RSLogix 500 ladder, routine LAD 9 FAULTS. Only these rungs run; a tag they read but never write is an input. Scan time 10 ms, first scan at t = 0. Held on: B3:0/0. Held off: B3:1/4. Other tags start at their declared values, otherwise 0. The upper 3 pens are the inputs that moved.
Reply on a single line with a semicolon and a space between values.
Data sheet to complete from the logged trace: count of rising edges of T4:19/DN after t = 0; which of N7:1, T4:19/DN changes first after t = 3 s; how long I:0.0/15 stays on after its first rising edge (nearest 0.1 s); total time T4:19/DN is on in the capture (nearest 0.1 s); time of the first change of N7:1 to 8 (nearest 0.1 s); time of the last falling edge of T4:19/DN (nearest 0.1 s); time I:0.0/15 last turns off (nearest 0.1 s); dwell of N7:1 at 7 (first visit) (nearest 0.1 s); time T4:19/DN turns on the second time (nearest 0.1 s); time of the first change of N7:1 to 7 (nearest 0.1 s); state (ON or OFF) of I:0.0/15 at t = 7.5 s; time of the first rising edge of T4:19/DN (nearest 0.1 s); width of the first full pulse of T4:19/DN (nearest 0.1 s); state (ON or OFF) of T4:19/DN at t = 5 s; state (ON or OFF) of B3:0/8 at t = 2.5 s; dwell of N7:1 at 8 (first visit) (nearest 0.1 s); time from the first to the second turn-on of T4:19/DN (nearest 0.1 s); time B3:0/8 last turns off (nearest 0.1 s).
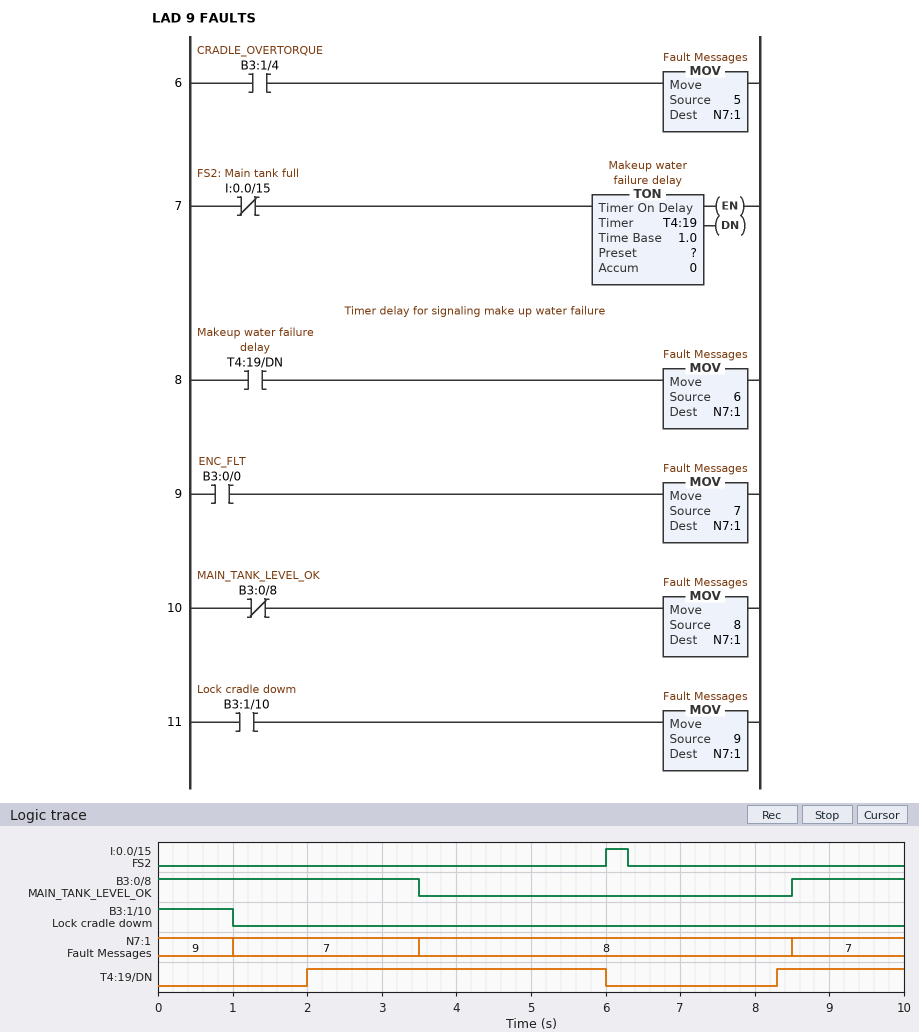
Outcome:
2; N7:1; 0.3 s; 5.7 s; 3.5 s; 6.0 s; 6.3 s; 2.5 s; 8.3 s; 1.0 s; OFF; 2.0 s; 4.0 s; ON; ON; 5.0 s; 6.3 s; 3.5 s
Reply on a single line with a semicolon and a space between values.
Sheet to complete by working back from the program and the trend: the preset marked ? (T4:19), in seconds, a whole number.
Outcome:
2 s
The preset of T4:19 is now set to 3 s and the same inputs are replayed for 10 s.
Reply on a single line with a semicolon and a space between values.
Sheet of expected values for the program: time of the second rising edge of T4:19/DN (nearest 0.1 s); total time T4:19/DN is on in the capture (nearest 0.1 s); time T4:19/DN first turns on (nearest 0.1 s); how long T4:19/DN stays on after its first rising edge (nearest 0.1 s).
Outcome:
9.3 s; 3.7 s; 3.0 s; 3.0 s
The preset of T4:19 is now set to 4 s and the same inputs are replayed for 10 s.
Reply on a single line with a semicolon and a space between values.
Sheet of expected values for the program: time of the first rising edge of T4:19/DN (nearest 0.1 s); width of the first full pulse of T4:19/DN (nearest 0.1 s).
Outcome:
4.0 s; 2.0 s
